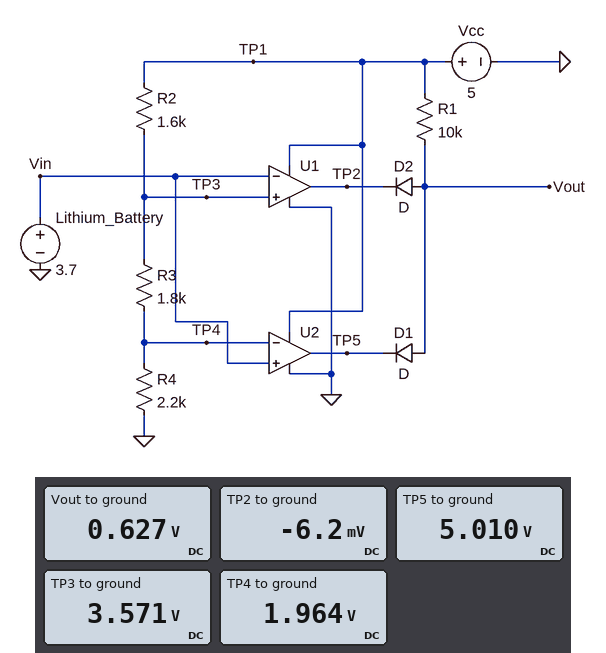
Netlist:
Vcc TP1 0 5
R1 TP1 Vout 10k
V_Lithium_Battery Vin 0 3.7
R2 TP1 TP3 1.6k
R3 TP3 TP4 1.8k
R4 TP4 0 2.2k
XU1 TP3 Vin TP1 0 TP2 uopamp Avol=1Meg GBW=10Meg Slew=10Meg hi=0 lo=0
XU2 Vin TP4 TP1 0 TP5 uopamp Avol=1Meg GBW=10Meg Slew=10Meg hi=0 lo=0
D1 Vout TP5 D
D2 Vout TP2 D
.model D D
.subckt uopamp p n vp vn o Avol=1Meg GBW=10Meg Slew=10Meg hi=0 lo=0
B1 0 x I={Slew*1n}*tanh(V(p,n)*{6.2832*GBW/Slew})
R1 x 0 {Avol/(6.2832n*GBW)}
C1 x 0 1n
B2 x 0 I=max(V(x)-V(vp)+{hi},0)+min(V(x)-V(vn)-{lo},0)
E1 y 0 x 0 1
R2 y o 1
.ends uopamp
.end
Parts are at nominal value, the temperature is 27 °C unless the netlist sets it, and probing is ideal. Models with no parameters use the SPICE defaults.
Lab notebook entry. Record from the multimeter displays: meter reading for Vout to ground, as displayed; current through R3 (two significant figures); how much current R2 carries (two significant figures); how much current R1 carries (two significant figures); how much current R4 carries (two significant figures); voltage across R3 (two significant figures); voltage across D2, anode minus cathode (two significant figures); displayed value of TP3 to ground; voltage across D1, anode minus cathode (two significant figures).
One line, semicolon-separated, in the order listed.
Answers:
0.627 V; 890 µA; 890 µA; 440 µA; 890 µA; 1.6 V; 630 mV; 3.571 V; -4.4 V
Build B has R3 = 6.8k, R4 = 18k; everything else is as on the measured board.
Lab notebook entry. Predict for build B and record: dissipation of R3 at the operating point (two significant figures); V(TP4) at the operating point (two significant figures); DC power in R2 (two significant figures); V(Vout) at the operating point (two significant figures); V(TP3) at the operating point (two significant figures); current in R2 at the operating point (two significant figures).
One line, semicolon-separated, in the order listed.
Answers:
240 µW; 3.4 V; 57 µW; 5.0 V; 4.7 V; 190 µA
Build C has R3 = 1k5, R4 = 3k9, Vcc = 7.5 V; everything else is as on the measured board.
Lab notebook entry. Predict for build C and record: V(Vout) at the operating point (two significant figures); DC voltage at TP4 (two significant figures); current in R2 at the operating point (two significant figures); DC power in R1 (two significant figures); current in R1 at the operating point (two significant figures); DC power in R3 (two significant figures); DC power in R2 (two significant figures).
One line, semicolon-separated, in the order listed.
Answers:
640 mV; 4.2 V; 1.1 mA; 4.7 mW; 690 µA; 1.7 mW; 1.8 mW
